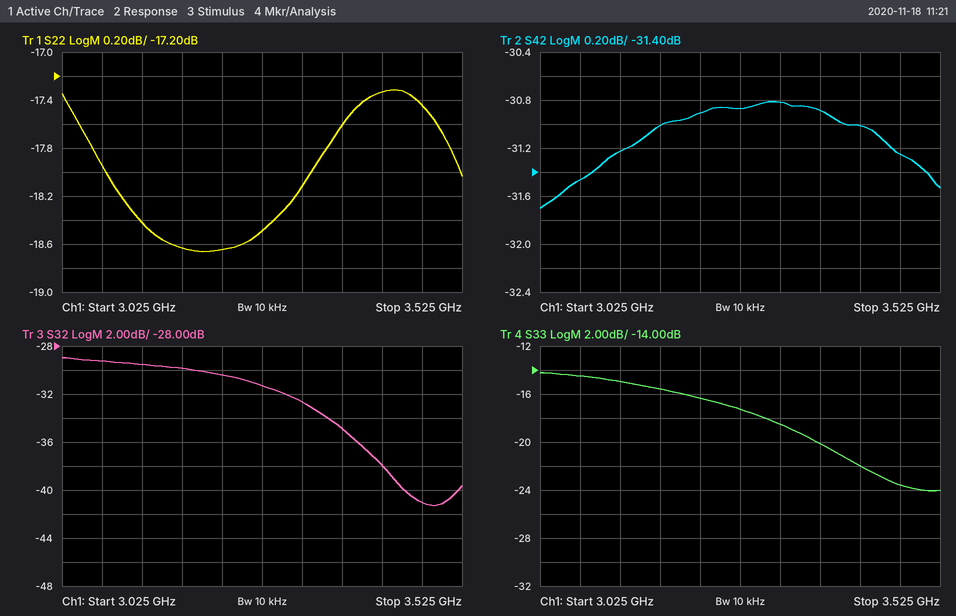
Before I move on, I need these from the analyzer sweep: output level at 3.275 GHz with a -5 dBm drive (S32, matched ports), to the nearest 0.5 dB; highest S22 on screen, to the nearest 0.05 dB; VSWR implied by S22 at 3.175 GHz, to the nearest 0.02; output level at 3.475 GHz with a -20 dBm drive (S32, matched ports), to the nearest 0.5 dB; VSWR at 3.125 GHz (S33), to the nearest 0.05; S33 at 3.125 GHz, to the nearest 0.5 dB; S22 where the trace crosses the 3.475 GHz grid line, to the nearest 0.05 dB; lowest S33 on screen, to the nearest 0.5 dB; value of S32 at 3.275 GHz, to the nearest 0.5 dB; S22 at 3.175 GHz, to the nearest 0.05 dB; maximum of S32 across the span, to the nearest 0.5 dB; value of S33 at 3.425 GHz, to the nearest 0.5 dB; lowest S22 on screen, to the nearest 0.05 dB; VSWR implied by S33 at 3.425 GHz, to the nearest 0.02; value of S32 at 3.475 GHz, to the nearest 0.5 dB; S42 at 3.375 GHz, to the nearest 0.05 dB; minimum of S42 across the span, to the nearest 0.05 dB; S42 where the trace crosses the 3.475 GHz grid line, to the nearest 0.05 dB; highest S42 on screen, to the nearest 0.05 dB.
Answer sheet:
-36.5 dBm
-17.30 dB
1.26
-61.0 dBm
1.45
-15.0 dB
-17.45 dB
-24.0 dB
-31.5 dB
-18.65 dB
-29.0 dB
-22.0 dB
-18.65 dB
1.18
-41.0 dB
-30.90 dB
-31.70 dB
-31.25 dB
-30.80 dB
